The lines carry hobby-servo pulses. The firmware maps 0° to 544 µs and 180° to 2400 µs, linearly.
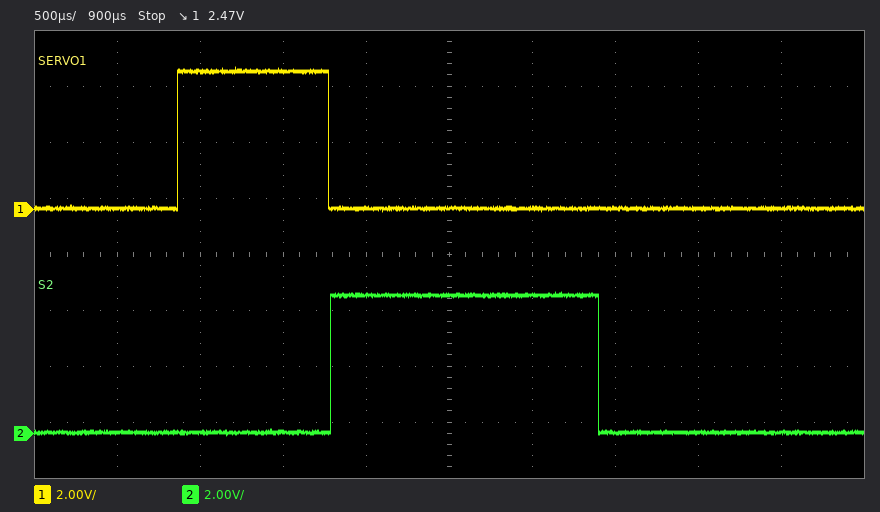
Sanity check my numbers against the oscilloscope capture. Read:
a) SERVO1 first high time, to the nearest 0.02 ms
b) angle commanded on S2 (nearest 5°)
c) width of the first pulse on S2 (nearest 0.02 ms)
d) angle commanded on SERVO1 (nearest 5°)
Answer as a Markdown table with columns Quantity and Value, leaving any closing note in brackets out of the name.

| Quantity | Value |
|---|---|
| SERVO1 first high time, to the nearest 0.02 ms | 0.92 ms |
| angle commanded on S2 | 105° |
| width of the first pulse on S2 | 1.62 ms |
| angle commanded on SERVO1 | 35° |
